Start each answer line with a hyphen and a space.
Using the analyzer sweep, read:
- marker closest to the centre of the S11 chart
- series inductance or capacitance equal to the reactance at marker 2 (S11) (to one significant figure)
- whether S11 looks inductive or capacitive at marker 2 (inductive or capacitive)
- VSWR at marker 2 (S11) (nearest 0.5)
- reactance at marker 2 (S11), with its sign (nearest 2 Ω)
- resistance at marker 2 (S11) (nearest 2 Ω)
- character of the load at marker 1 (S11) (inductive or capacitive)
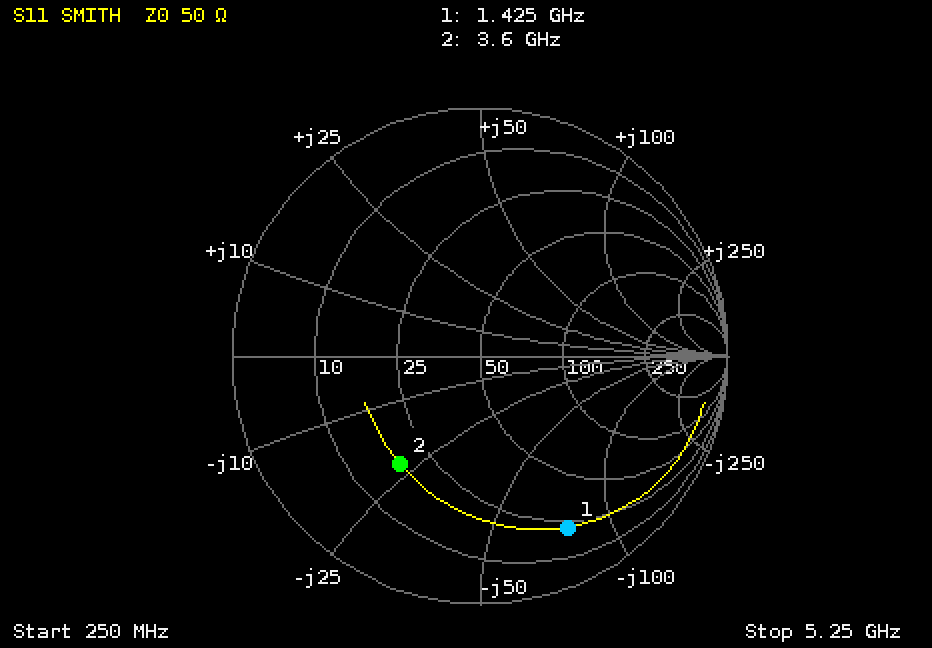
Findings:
- marker 2
- 2 pF
- capacitive
- 3.5
- -22 Ω
- 18 Ω
- capacitive
